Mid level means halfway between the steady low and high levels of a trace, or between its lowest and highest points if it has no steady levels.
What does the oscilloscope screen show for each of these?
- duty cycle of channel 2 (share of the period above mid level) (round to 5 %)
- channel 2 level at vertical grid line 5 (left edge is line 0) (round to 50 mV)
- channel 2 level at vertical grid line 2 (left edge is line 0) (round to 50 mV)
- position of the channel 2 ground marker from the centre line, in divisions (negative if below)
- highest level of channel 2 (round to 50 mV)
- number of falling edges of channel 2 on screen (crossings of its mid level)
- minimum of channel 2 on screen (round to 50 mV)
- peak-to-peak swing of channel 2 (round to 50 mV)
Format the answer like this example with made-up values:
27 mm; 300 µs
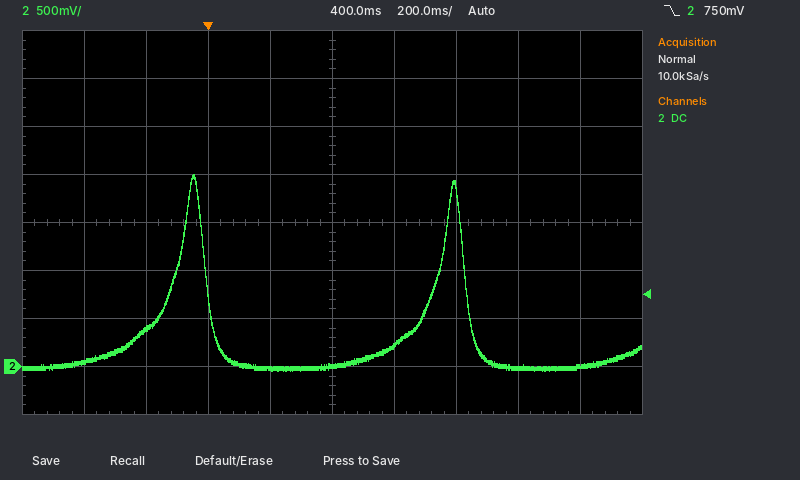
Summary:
10 %; 0 mV; 400 mV; -3.0 div; 2.00 V; 2; -50 mV; 2.05 V
